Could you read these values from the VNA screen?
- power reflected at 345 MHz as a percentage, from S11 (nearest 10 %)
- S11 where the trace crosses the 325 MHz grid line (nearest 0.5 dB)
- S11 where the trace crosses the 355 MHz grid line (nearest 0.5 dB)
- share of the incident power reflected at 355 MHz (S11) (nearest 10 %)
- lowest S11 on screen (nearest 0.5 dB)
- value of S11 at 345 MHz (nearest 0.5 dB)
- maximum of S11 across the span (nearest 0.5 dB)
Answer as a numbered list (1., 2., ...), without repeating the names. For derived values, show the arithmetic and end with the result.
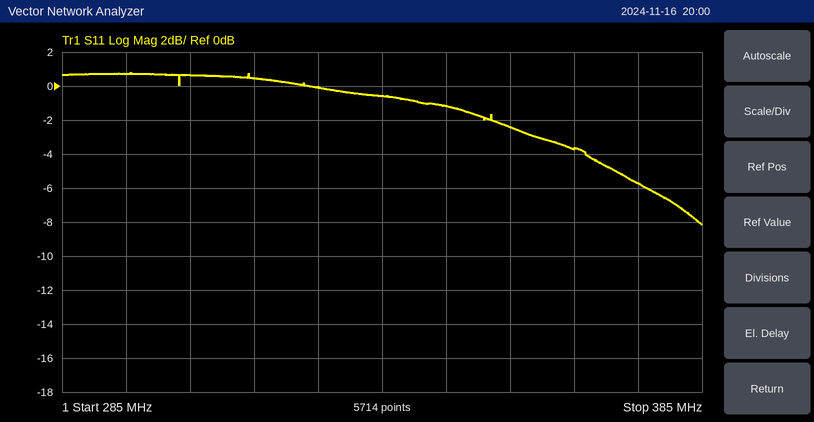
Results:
1. 10^(-1/10) ≈ 79.4 %, so 80 % to the nearest 10 %
2. 0.0 dB
3. -2.5 dB
4. 10^(-2.5/10) ≈ 56.2 %, so 60 % to the nearest 10 %
5. -8.0 dB
6. -1.0 dB
7. 1.0 dB
